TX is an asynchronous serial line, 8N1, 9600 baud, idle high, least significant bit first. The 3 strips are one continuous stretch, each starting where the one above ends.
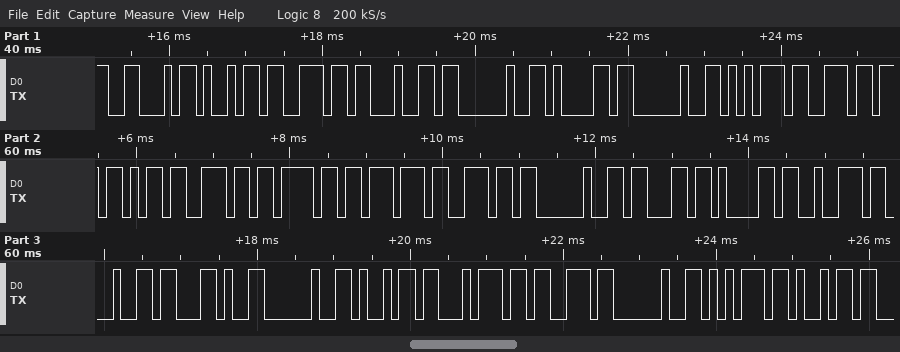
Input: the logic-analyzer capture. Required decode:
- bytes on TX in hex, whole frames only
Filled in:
0x46 0x69 0x6E 0x64 0x20 0x61 0x20 0x75 0x6E 0x6B 0x6E 0x6F 0x77 0x6E 0x20 0x63 0x61 0x72 0x64 0x2C 0x20 0x69 0x74 0x73 0x20 0x75 0x69
